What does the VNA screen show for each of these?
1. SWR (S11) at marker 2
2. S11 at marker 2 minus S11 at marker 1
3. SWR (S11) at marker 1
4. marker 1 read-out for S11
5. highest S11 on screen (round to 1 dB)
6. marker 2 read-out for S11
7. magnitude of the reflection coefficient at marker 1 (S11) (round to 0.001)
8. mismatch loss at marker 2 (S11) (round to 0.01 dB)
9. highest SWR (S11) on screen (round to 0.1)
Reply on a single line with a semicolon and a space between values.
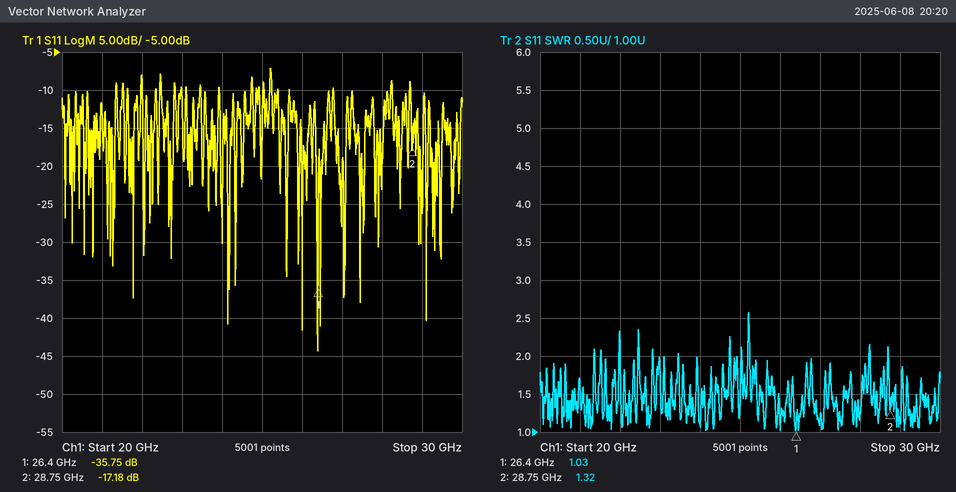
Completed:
1.32; 18.57 dB; 1.03; -35.75 dB; -7 dB; -17.18 dB; 0.016; 0.08 dB; 2.6
